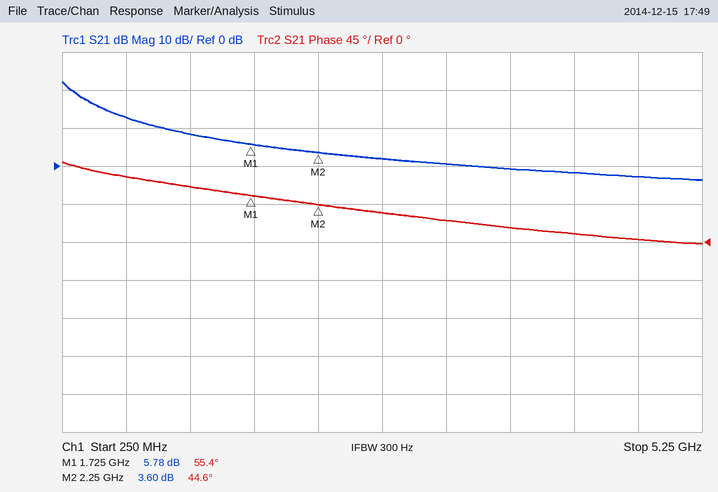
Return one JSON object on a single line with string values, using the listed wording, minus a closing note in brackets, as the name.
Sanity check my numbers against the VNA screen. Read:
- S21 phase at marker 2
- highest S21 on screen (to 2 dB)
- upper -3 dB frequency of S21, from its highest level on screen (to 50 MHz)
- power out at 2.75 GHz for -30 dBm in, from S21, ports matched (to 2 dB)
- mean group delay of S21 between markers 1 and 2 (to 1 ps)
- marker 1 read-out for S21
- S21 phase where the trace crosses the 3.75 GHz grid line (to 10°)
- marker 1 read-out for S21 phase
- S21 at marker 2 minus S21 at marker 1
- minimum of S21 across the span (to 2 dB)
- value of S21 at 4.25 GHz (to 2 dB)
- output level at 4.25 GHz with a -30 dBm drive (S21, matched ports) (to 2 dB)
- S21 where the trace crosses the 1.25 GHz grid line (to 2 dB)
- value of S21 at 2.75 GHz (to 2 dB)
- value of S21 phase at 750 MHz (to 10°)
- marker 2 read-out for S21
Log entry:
{"S21 phase at marker 2": "44.6°", "highest S21 on screen": "22 dB", "upper -3 dB frequency of S21, from its highest level on screen": "350 MHz", "power out at 2.75 GHz for -30 dBm in, from S21, ports matched": "-28 dBm", "mean group delay of S21 between markers 1 and 2": "57 ps", "marker 1 read-out for S21": "5.78 dB", "S21 phase where the trace crosses the 3.75 GHz grid line": "20°", "marker 1 read-out for S21 phase": "55.4°", "S21 at marker 2 minus S21 at marker 1": "-2.18 dB", "minimum of S21 across the span": "-4 dB", "value of S21 at 4.25 GHz": "-2 dB", "output level at 4.25 GHz with a -30 dBm drive (S21, matched ports)": "-32 dBm", "S21 where the trace crosses the 1.25 GHz grid line": "8 dB", "value of S21 at 2.75 GHz": "2 dB", "value of S21 phase at 750 MHz": "80°", "marker 2 read-out for S21": "3.60 dB"}
